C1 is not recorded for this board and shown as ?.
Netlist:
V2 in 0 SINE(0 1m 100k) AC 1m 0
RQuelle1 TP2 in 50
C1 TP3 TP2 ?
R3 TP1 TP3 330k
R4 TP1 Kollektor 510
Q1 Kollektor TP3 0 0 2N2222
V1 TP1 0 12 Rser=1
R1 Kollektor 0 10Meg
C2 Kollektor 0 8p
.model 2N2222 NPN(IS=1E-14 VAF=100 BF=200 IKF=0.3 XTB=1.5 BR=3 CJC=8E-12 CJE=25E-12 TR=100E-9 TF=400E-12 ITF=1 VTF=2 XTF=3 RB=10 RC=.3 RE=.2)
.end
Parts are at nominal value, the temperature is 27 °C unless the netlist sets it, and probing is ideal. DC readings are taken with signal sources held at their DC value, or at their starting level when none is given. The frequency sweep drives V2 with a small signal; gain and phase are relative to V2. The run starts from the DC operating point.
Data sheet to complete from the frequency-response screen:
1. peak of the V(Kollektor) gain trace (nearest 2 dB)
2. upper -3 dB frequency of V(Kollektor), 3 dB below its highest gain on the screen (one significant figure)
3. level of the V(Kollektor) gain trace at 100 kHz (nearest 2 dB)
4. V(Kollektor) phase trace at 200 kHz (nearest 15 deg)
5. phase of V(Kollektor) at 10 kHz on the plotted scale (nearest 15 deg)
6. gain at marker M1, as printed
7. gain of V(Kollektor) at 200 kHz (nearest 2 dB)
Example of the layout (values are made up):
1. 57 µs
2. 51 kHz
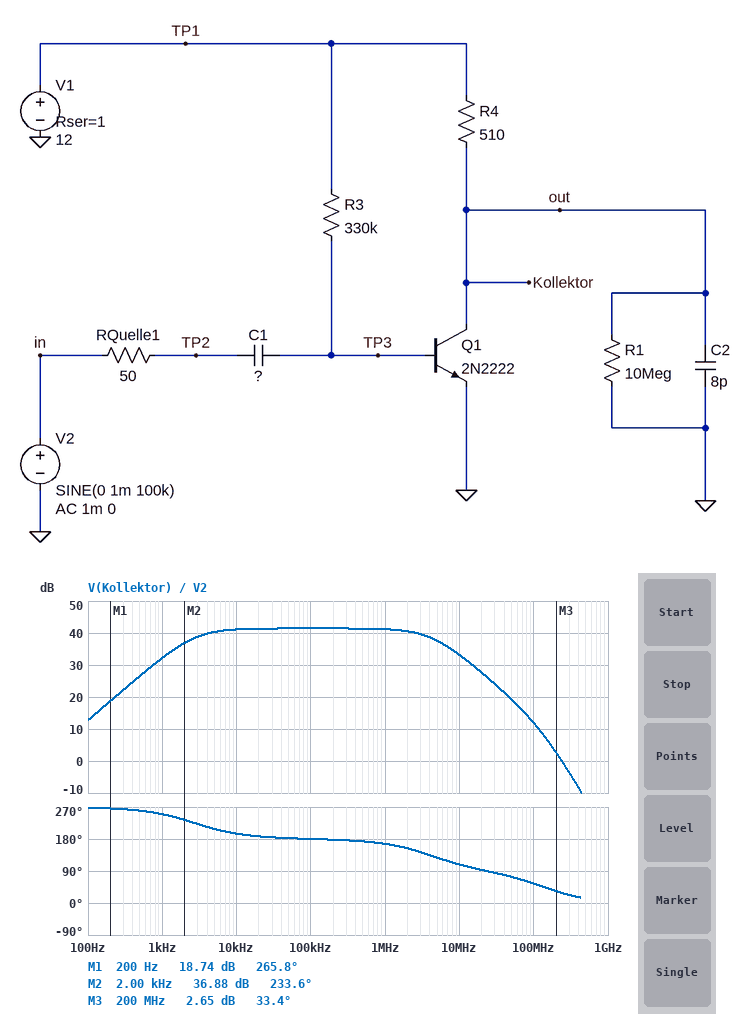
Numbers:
1. 42 dB
2. 4 MHz
3. 42 dB
4. 180 deg
5. 195 deg
6. 18.74 dB
7. 42 dB
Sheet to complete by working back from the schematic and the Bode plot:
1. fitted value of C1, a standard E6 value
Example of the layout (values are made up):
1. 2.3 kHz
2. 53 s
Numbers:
1. 68 nF
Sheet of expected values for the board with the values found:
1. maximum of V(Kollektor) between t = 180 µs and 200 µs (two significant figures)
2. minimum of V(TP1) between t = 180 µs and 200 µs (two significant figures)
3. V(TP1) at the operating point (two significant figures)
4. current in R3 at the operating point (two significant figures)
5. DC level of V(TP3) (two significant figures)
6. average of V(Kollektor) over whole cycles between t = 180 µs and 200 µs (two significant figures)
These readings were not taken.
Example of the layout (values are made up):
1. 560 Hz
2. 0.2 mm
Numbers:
1. 8.4 V
2. 12 V
3. 12 V
4. 34 µA
5. 710 mV
6. 8.3 V
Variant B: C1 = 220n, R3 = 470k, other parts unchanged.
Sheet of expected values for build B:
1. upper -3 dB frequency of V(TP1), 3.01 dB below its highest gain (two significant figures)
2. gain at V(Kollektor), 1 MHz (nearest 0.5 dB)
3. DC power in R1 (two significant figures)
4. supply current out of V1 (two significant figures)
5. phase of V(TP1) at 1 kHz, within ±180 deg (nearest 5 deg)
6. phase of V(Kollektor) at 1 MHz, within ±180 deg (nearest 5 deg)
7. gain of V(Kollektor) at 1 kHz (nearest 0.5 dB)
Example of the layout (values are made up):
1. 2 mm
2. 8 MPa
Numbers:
1. 5.4 MHz
2. 39.0 dB
3. 8.8 µW
4. 5.2 mA
5. -150 deg
6. 170 deg
7. 37.5 dB
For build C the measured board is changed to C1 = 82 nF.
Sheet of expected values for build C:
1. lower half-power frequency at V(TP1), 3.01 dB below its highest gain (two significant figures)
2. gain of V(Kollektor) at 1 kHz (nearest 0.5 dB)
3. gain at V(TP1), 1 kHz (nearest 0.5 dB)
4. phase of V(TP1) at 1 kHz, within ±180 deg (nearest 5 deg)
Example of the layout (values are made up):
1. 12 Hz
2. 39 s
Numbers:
1. 2.3 kHz
2. 33.5 dB
3. -20.5 dB
4. -115 deg
